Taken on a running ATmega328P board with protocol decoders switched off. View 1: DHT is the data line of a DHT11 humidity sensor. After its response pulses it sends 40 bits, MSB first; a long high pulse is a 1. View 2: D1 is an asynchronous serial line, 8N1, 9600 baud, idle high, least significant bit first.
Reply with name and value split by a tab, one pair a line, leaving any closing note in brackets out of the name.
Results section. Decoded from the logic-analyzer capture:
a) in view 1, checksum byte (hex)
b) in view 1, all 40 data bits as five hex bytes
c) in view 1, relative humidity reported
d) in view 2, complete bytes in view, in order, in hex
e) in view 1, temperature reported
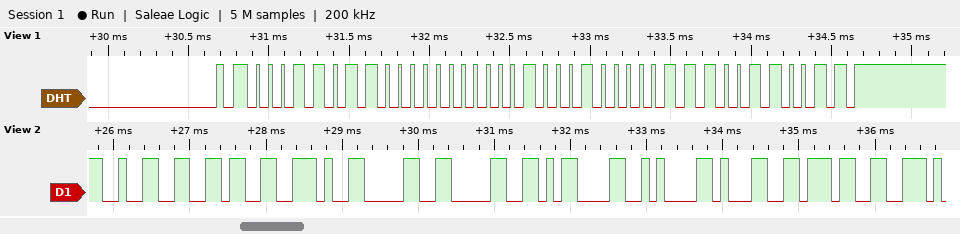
in view 1, checksum byte	0x33
in view 1, all 40 data bits as five hex bytes	1B 00 11 07 33
in view 1, relative humidity reported	27 %
in view 2, complete bytes in view, in order, in hex	32 36 2E 30 30 0D 0A 31 37
in view 1, temperature reported	17.7 °C
